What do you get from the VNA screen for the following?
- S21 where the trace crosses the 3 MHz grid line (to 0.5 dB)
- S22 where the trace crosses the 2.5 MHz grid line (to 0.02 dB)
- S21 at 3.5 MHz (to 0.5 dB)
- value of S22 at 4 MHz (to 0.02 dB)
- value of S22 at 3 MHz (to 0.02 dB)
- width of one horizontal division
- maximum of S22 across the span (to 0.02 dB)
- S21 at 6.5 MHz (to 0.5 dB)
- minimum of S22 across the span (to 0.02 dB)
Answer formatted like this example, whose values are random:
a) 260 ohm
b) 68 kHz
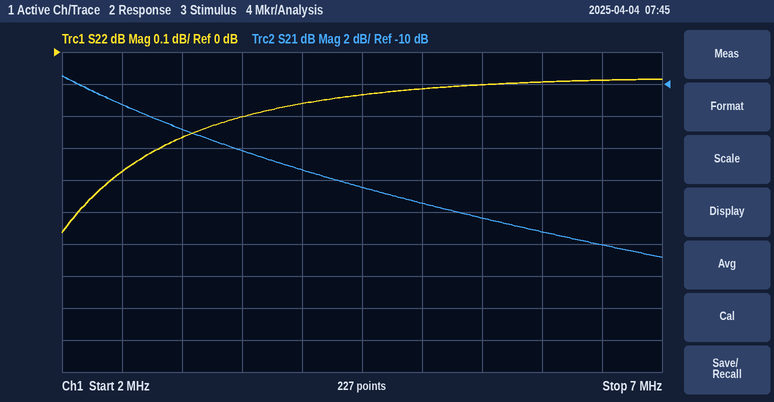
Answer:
a) -13.0 dB
b) -0.38 dB
c) -14.0 dB
d) -0.16 dB
e) -0.26 dB
f) 500 kHz
g) -0.08 dB
h) -20.0 dB
i) -0.56 dB
